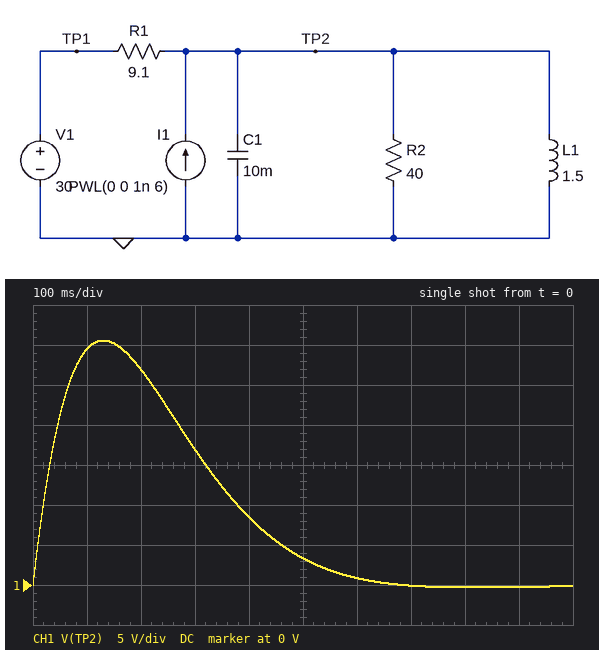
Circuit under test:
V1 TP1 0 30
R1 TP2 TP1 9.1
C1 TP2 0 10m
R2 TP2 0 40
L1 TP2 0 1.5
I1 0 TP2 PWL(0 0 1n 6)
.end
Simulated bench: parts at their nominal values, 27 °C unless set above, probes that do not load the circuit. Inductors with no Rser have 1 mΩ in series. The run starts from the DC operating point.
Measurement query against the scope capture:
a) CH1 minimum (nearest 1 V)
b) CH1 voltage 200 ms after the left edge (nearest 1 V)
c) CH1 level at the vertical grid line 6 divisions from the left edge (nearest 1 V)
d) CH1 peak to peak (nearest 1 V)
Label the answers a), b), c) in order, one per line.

a) 0 V
b) 27 V
c) 1 V
d) 31 V
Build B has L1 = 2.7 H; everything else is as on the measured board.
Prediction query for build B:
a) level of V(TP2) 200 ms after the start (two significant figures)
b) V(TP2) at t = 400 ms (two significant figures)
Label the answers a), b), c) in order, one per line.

a) 33 V
b) 20 V
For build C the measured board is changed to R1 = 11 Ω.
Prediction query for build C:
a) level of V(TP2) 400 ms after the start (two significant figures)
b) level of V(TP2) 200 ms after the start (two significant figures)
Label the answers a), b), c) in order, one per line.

a) 7.7 V
b) 30 V
